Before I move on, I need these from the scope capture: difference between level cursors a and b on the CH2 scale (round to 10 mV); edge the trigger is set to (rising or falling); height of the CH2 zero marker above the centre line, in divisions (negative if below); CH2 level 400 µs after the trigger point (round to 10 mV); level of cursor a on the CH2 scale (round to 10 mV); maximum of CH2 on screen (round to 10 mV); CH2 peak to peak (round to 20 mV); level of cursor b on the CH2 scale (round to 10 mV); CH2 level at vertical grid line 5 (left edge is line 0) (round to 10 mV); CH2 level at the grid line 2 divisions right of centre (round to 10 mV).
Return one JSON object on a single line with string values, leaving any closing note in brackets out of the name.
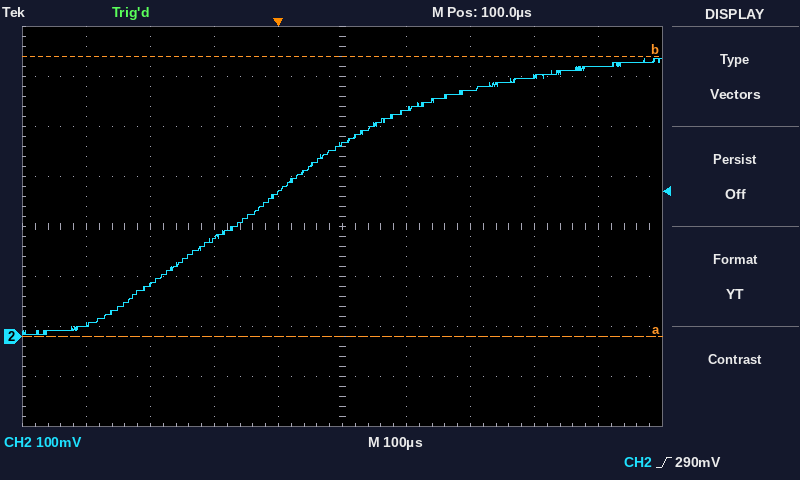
{"difference between level cursors a and b on the CH2 scale": "560 mV", "edge the trigger is set to": "rising", "height of the CH2 zero marker above the centre line, in divisions": "-2.2 div", "CH2 level 400 µs after the trigger point": "520 mV", "level of cursor a on the CH2 scale": "0 mV", "maximum of CH2 on screen": "560 mV", "CH2 peak to peak": "560 mV", "level of cursor b on the CH2 scale": "560 mV", "CH2 level at vertical grid line 5 (left edge is line 0)": "380 mV", "CH2 level at the grid line 2 divisions right of centre": "490 mV"}
